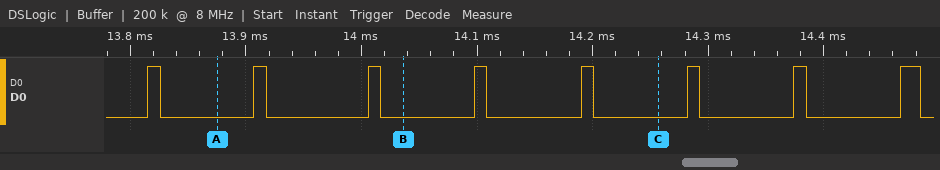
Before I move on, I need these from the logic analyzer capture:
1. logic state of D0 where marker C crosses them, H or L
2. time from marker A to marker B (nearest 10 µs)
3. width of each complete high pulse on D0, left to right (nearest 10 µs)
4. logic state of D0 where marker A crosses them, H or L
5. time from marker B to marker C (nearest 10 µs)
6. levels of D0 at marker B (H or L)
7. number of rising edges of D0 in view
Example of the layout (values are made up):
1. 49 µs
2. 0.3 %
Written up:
1. D0=L
2. 160 µs
3. 10 µs, 10 µs, 10 µs, 10 µs, 10 µs, 10 µs, 10 µs, 20 µs
4. D0=L
5. 220 µs
6. D0=L
7. 8
